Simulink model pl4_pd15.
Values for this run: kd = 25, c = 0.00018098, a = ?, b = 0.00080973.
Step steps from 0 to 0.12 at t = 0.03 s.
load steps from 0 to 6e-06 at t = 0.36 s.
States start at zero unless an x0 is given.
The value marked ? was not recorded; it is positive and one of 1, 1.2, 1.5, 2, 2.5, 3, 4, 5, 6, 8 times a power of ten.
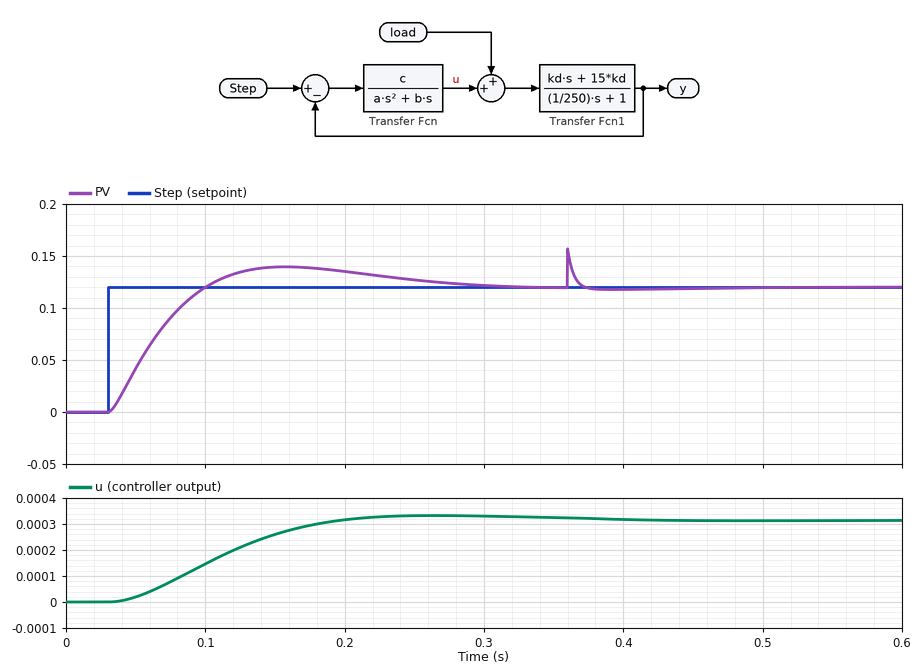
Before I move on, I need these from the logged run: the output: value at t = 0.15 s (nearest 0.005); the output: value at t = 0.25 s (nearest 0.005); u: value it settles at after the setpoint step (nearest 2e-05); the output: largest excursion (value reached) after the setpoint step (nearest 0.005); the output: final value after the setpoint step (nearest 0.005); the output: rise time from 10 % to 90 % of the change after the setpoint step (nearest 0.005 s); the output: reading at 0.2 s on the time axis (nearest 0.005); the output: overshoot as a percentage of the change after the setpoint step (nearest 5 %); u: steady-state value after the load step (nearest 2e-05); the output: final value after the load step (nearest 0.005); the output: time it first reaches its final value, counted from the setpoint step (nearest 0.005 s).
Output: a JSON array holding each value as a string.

["0.140", "0.125", "0.00032", "0.140", "0.120", "0.050 s", "0.135", "15 %", "0.00032", "0.120", "0.070 s"]
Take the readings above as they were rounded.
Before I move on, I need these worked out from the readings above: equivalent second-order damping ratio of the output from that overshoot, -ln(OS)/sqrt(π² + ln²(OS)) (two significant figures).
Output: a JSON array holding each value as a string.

["0.52"]
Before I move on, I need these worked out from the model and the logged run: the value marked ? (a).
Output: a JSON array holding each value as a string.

["0.0002"]
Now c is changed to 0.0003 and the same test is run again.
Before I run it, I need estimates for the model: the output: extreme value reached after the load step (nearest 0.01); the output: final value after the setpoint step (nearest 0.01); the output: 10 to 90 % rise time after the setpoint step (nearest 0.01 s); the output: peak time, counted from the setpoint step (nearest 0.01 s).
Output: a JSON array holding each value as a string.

["0.16", "0.12", "0.03 s", "0.09 s"]
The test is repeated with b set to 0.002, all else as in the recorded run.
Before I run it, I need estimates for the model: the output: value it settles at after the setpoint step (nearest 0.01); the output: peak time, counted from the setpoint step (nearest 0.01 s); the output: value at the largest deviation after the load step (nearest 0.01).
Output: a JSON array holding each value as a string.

["0.12", "0.15 s", "0.16"]
